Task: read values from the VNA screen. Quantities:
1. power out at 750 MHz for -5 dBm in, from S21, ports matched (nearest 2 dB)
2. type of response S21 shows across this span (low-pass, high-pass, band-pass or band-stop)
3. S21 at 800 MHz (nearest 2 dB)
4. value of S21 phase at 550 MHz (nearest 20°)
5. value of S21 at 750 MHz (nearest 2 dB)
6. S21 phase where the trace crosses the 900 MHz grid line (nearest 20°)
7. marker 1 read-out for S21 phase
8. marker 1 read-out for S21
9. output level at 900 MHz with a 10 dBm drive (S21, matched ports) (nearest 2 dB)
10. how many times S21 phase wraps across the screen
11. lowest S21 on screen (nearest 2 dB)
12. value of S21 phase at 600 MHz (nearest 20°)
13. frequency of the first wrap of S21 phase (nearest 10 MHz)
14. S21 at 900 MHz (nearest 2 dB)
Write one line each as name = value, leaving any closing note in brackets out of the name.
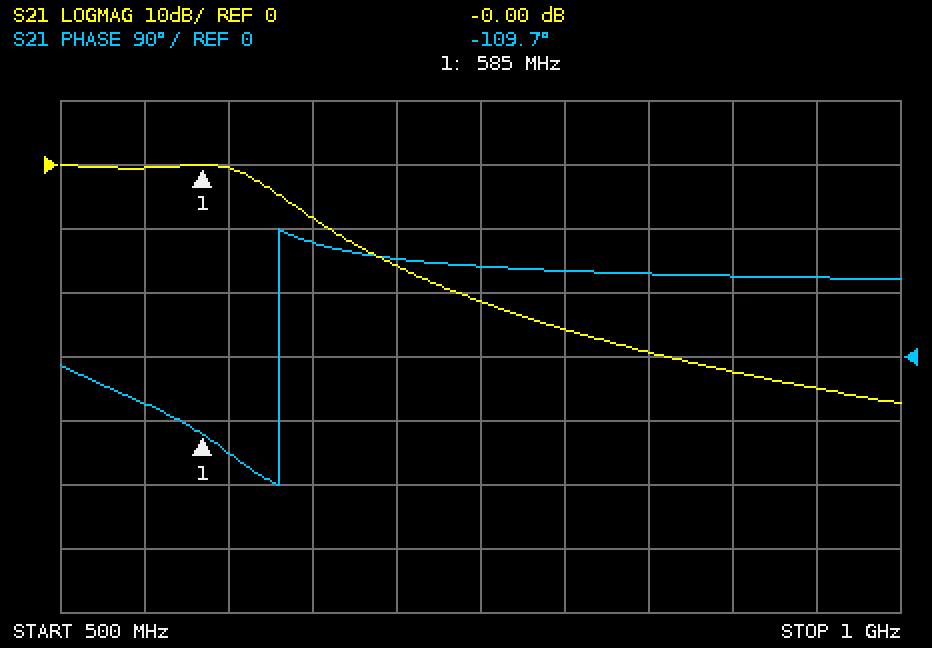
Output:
power out at 750 MHz for -5 dBm in, from S21, ports matched = -26 dBm
type of response S21 shows across this span = low-pass
S21 at 800 MHz = -26 dB
value of S21 phase at 550 MHz = -60°
value of S21 at 750 MHz = -22 dB
S21 phase where the trace crosses the 900 MHz grid line = 120°
marker 1 read-out for S21 phase = -109.7°
marker 1 read-out for S21 = -0.00 dB
output level at 900 MHz with a 10 dBm drive (S21, matched ports) = -22 dBm
how many times S21 phase wraps across the screen = 1
lowest S21 on screen = -38 dB
value of S21 phase at 600 MHz = -140°
frequency of the first wrap of S21 phase = 630 MHz
S21 at 900 MHz = -32 dB
